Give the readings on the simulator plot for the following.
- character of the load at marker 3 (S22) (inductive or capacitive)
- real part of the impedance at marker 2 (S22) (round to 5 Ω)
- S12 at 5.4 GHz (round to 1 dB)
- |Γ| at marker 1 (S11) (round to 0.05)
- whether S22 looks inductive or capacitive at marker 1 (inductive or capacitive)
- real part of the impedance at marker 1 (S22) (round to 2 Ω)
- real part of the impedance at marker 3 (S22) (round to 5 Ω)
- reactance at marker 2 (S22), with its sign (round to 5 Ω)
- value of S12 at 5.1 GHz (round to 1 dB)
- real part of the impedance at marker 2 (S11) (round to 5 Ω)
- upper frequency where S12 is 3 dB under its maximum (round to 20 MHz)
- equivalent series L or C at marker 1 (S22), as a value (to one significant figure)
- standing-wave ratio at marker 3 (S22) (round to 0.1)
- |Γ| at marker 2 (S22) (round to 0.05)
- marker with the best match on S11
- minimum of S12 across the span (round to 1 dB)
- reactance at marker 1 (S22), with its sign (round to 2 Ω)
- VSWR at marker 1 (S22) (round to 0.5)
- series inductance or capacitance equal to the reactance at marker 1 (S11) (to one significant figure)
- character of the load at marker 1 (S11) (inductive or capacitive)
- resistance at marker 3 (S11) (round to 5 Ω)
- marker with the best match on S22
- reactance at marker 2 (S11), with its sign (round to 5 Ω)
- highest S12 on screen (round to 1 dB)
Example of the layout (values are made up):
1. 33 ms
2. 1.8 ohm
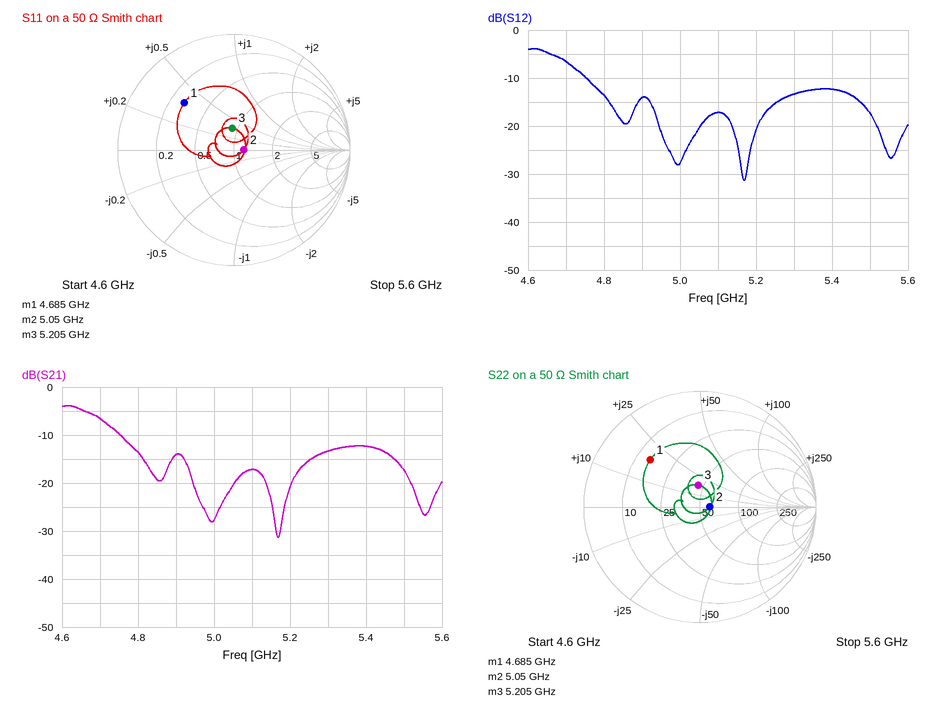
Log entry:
1. inductive
2. 60 Ω
3. -12 dB
4. 0.60
5. inductive
6. 14 Ω
7. 45 Ω
8. 0 Ω
9. -17 dB
10. 60 Ω
11. 4.70 GHz
12. 600 pH
13. 1.5
14. 0.10
15. marker 2
16. -31 dB
17. +18 Ω
18. 4.0
19. 600 pH
20. inductive
21. 45 Ω
22. marker 2
23. 0 Ω
24. -4 dB
